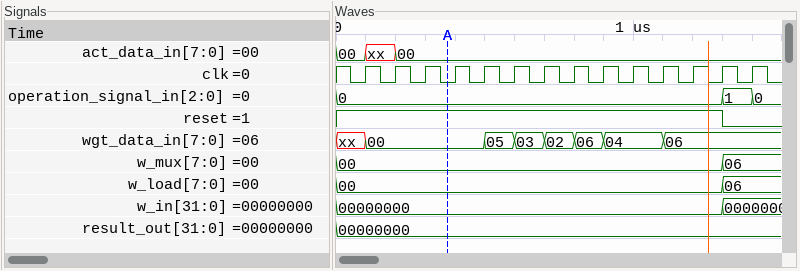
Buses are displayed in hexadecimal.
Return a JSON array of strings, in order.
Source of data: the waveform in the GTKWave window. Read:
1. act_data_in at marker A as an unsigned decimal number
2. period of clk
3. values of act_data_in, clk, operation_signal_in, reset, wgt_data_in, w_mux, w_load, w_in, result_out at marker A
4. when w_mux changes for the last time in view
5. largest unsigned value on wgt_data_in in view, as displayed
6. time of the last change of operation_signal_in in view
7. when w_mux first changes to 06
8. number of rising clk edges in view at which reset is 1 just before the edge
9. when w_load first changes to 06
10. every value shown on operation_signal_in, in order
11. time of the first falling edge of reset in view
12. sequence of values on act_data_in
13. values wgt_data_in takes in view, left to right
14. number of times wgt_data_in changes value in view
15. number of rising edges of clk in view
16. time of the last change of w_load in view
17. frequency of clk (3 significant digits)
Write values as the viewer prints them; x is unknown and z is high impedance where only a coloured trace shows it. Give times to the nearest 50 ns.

["0", "100 ns", "act_data_in=00, clk=0, operation_signal_in=0, reset=1, wgt_data_in=00, w_mux=00, w_load=00, w_in=00000000, result_out=00000000", "1300 ns", "06", "1400 ns", "1300 ns", "13", "1300 ns", "0, 1, 0", "1300 ns", "00, xx, 00", "xx, 00, 05, 03, 02, 06, 04, 06", "7", "14", "1300 ns", "10.0 MHz"]
